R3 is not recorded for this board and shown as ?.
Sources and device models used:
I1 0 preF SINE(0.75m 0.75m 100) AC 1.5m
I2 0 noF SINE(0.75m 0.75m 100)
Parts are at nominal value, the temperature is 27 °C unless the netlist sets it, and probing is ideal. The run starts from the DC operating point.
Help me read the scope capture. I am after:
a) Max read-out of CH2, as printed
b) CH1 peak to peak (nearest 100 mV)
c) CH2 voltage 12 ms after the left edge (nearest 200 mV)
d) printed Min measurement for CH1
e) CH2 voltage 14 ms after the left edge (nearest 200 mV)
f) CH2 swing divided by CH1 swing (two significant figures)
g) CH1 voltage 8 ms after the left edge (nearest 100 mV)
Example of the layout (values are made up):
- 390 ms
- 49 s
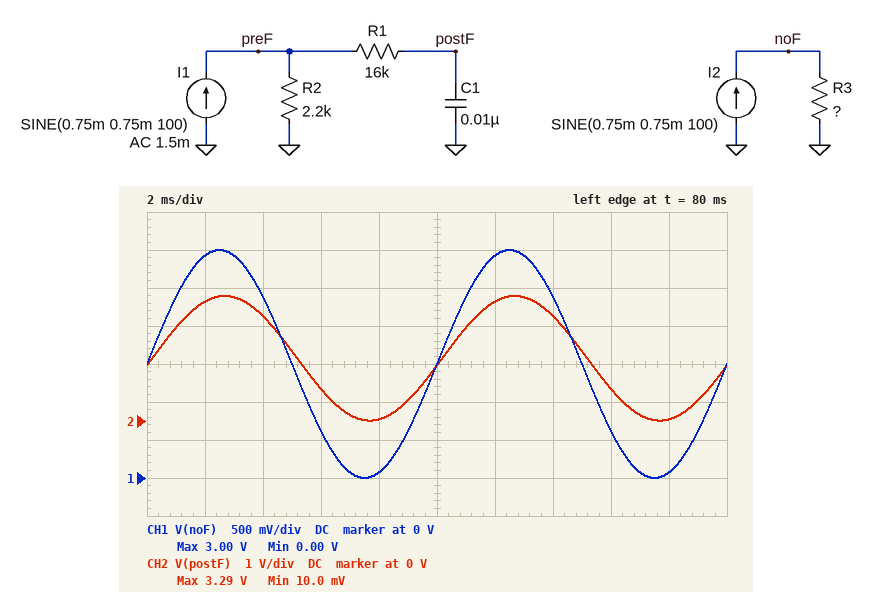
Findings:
- 3.29 V
- 3.0 V
- 3.2 V
- 0.00 V
- 2.8 V
- 1.1
- 100 mV
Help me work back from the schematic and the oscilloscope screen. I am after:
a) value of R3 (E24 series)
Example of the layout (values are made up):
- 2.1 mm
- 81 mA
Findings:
- 2 kΩ
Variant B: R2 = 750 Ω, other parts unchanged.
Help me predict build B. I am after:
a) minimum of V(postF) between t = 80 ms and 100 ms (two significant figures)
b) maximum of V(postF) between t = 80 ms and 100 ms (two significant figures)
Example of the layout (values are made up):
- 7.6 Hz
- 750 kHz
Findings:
- 3.1 mV
- 1.1 V
